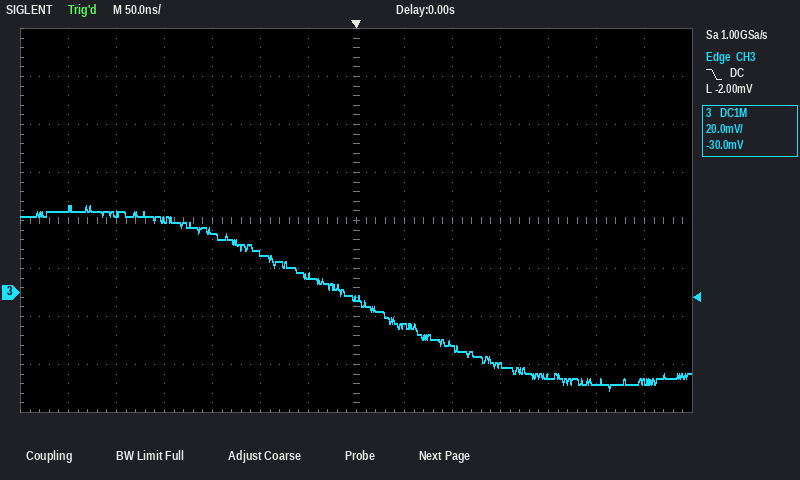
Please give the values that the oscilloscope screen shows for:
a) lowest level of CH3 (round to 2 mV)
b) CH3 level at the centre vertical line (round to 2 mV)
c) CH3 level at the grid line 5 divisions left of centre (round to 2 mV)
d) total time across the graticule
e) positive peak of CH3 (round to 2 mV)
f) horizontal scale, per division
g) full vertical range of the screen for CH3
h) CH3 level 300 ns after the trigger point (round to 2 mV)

-40 mV
-2 mV
32 mV
700 ns
36 mV
50 ns
160 mV
-38 mV
